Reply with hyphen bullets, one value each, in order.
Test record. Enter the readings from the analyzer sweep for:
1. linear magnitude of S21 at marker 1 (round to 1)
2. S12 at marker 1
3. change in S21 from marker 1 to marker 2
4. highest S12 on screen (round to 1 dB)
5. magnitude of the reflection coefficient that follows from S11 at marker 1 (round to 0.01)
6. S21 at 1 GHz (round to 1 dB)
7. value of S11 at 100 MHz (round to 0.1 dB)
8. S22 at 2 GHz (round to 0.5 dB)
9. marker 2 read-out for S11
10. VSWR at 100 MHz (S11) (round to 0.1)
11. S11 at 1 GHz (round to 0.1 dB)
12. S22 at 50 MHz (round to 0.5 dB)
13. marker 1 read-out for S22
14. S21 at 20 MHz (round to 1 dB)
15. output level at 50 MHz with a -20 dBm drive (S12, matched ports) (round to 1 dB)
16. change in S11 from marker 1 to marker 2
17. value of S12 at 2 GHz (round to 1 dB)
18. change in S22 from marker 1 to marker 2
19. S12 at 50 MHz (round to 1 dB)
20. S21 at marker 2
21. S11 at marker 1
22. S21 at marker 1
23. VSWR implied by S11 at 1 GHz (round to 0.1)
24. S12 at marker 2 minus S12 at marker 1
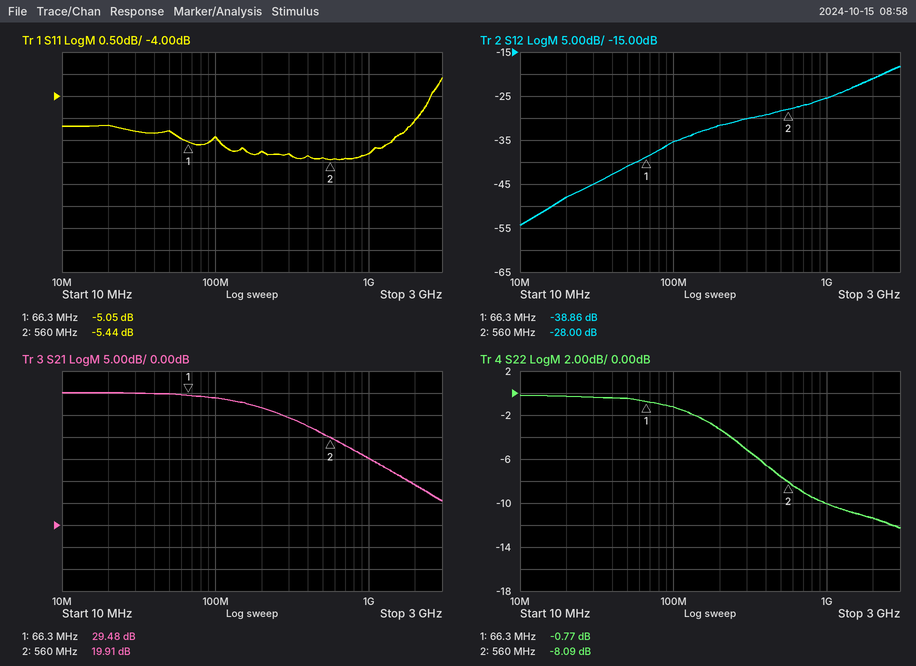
- 30
- -38.86 dB
- -9.57 dB
- -18 dB
- 0.56
- 15 dB
- -4.9 dB
- -11.5 dB
- -5.44 dB
- 3.6
- -5.3 dB
- -0.5 dB
- -0.77 dB
- 30 dB
- -61 dBm
- -0.39 dB
- -21 dB
- -7.32 dB
- -41 dB
- 19.91 dB
- -5.05 dB
- 29.48 dB
- 3.4
- 10.86 dB
